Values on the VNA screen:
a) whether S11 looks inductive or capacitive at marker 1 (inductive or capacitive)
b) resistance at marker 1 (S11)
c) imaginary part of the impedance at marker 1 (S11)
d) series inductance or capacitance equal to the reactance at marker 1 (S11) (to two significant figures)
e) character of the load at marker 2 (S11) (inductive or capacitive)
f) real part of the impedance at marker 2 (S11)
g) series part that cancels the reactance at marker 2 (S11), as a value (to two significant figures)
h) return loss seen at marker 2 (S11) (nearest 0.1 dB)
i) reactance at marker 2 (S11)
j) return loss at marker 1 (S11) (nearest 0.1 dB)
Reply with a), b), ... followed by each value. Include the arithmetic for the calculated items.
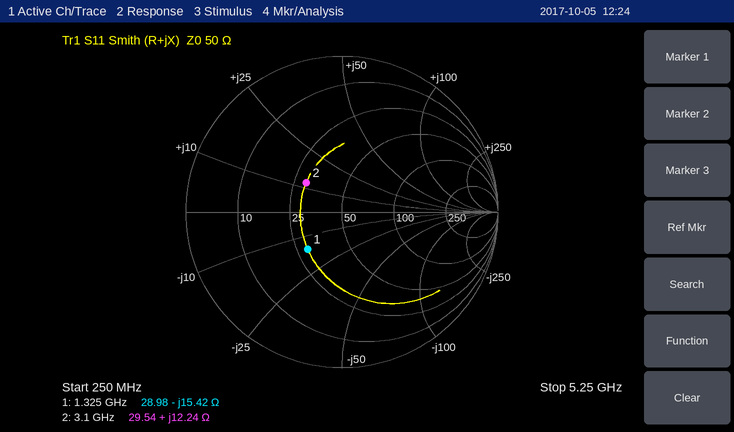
a) capacitive
b) 28.98 Ω
c) -15.42 Ω
d) C = 1/(2π × 1.325 GHz × 15.42 Ω) ≈ 7.8 pF
e) inductive
f) 29.54 Ω
g) C = 1/(2π × 3.1 GHz × 12.24 Ω) ≈ 4.2 pF
h) 10.6 dB
i) +12.24 Ω
j) 9.8 dB
